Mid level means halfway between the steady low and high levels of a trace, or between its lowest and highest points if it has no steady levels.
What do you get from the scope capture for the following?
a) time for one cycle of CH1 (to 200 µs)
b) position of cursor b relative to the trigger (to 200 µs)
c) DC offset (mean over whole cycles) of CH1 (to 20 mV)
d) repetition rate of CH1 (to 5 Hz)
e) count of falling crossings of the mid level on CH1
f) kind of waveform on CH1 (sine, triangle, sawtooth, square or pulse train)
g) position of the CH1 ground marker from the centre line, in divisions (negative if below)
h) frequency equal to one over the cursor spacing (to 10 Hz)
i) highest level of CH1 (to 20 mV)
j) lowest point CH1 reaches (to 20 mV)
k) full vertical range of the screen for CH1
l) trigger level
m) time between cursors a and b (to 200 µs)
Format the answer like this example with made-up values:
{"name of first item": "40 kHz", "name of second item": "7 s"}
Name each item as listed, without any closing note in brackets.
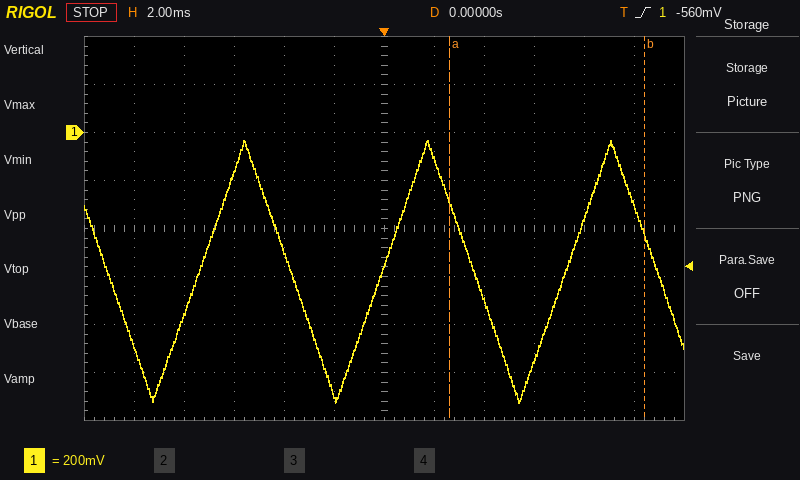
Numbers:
{"time for one cycle of CH1": "7.4 ms", "position of cursor b relative to the trigger": "+10.4 ms", "DC offset (mean over whole cycles) of CH1": "-580 mV", "repetition rate of CH1": "135 Hz", "count of falling crossings of the mid level on CH1": "4", "kind of waveform on CH1": "triangle", "position of the CH1 ground marker from the centre line, in divisions": "+2.0 div", "frequency equal to one over the cursor spacing": "130 Hz", "highest level of CH1": "-40 mV", "lowest point CH1 reaches": "-1.12 V", "full vertical range of the screen for CH1": "1.6 V", "trigger level": "-560 mV", "time between cursors a and b": "7.8 ms"}
